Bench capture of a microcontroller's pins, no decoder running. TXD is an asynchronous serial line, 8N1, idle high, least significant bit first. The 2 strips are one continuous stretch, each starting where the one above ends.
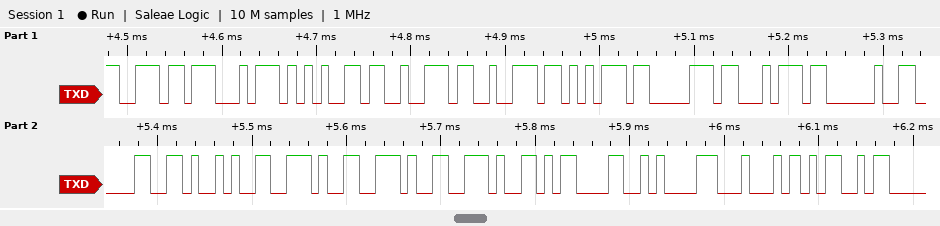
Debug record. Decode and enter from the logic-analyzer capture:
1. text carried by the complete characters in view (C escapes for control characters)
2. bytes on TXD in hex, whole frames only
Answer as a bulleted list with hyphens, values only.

- "nterrupt 0)...\r\nDM"
- 6E 74 65 72 72 75 70 74 20 30 29 2E 2E 2E 0D 0A 44 4D
